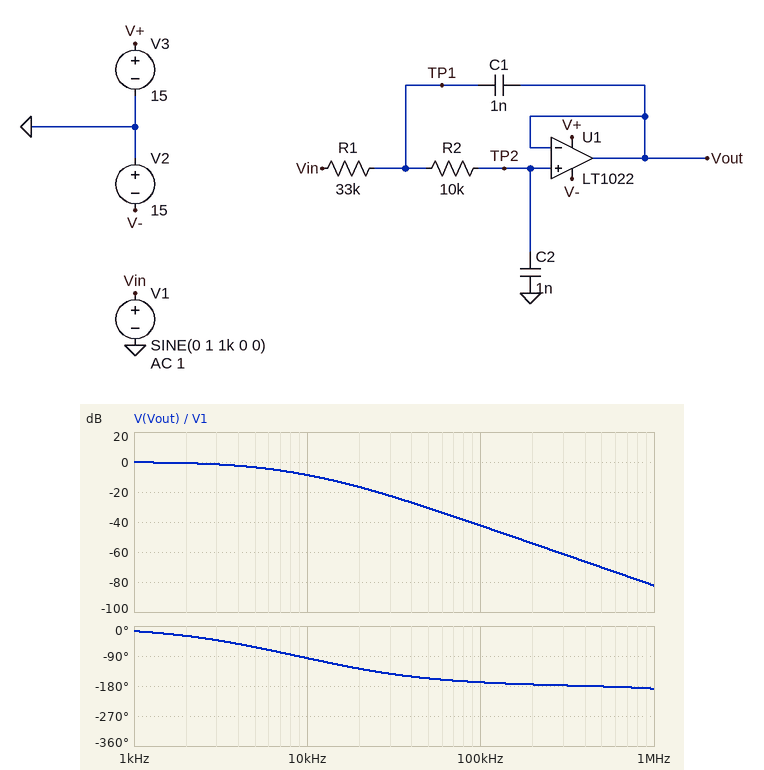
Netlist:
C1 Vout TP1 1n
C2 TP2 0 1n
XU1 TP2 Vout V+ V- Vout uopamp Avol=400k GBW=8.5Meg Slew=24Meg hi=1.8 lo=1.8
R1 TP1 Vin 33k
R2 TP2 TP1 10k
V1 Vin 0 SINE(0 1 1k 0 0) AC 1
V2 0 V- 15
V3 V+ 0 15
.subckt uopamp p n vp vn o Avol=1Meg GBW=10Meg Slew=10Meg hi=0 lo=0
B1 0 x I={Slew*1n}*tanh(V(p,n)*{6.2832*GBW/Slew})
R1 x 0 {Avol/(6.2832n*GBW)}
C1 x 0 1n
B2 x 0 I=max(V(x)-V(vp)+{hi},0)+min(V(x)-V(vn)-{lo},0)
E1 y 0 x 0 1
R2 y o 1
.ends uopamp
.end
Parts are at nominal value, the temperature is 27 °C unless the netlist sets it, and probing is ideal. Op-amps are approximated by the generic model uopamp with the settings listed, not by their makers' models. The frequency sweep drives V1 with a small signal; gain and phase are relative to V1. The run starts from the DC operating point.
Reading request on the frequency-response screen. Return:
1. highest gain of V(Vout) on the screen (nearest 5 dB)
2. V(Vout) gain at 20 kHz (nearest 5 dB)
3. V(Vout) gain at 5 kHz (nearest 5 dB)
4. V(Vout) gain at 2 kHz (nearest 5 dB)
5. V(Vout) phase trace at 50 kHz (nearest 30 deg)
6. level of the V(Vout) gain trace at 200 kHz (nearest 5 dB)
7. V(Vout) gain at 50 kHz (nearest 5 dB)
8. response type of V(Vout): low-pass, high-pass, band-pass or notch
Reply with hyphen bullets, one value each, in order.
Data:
- 0 dB
- -15 dB
- -5 dB
- 0 dB
- -150 deg
- -55 dB
- -30 dB
- low-pass
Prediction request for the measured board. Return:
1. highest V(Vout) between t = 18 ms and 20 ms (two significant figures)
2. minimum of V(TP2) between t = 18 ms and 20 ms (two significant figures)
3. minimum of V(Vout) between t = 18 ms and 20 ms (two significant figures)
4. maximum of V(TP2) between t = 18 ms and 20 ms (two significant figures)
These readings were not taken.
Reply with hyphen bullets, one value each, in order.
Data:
- 980 mV
- -980 mV
- -980 mV
- 980 mV
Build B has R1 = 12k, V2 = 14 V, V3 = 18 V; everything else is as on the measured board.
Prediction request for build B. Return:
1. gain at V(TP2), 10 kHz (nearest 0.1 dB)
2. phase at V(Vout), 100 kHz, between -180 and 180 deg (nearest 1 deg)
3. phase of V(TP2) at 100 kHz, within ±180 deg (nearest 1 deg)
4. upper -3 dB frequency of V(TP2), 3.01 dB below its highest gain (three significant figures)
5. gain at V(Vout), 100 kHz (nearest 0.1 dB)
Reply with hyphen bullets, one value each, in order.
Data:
- -3.4 dB
- -164 deg
- -163 deg
- 9.30 kHz
- -33.7 dB
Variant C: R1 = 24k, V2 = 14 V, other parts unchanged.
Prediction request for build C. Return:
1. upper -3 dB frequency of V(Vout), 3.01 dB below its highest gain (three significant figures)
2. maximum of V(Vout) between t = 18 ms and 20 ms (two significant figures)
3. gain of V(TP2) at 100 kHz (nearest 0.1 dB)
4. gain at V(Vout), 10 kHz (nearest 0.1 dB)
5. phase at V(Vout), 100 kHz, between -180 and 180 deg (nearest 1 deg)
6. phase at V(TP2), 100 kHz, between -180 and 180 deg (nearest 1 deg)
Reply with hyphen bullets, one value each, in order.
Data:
- 5.80 kHz
- 990 mV
- -39.7 dB
- -6.6 dB
- -168 deg
- -167 deg
